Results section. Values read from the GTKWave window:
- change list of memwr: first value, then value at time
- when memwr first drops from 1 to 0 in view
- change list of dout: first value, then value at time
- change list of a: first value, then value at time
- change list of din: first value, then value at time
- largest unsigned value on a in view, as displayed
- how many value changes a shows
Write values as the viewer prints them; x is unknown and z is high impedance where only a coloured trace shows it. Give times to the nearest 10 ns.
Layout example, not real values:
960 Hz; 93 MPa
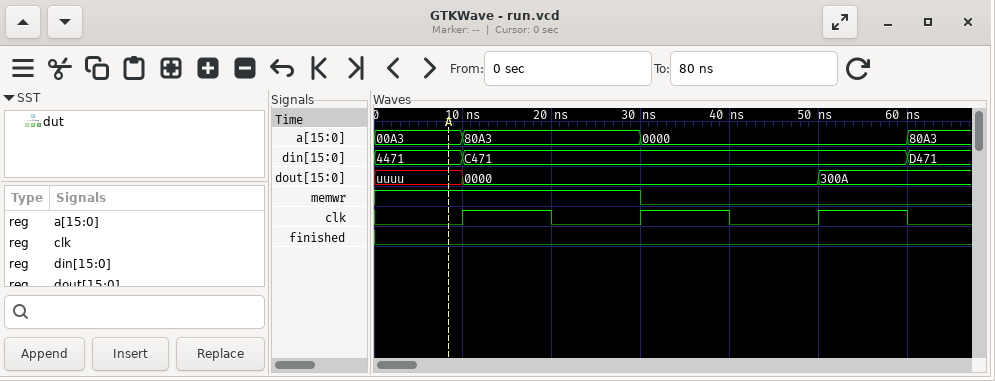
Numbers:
1, 0 at 30 ns; 30 ns; uuuu, 0000 at 10 ns, 300A at 50 ns; 00A3, 80A3 at 10 ns, 0000 at 30 ns, 80A3 at 60 ns; 4471, C471 at 10 ns, D471 at 60 ns; 80A3; 3
